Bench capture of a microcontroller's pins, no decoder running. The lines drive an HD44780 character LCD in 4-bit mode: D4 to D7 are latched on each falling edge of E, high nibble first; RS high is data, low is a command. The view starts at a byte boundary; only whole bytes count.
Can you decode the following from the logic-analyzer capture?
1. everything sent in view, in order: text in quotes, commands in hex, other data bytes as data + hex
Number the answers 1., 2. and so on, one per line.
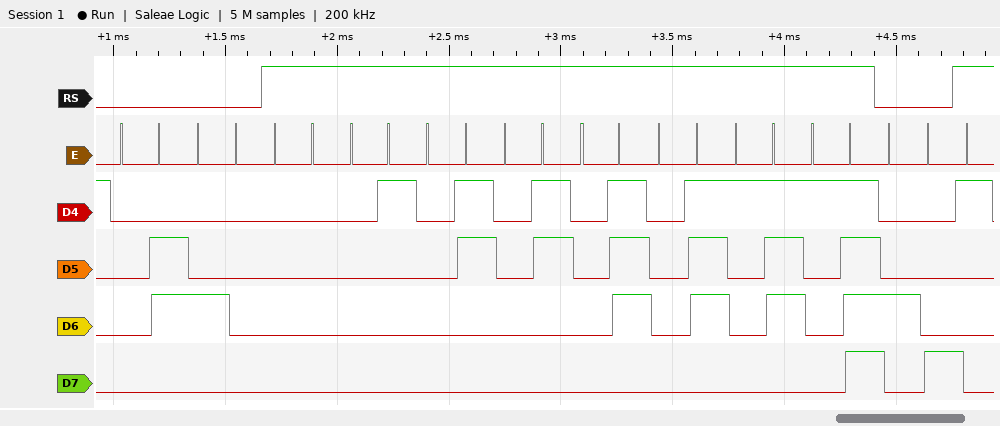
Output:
1. 0x06 0x40 data 00 01 03 03 07 07 17 1F 0x48
